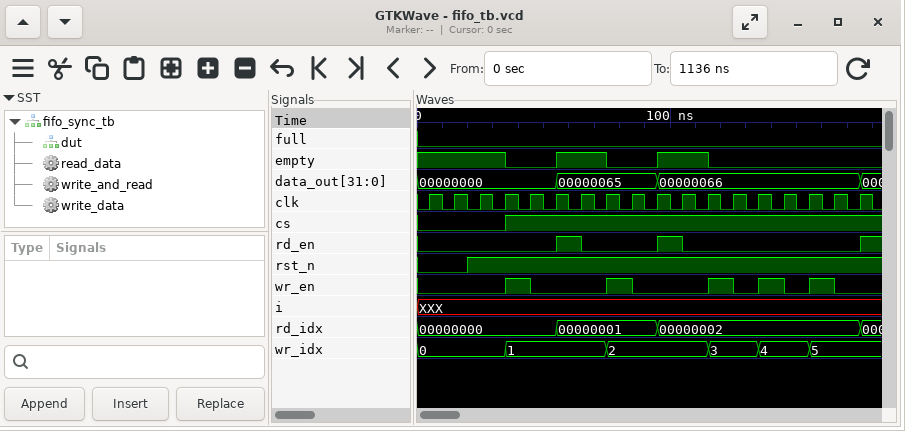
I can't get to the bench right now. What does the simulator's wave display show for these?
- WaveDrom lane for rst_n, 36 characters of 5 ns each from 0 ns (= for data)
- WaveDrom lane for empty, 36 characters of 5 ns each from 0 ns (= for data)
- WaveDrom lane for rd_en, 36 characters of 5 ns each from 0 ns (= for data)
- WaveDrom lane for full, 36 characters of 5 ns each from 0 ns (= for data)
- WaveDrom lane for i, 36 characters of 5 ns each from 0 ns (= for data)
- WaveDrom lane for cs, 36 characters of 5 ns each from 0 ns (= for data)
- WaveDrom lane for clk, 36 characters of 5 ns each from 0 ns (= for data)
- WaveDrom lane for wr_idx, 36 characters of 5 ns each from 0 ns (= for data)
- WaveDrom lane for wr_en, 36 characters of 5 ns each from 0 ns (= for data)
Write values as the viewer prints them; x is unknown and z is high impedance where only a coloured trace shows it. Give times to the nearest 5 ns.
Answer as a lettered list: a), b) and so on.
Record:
a) {name: 'rst_n', wave: '0...1...............................'}
b) {name: 'empty', wave: '1......0...1...0...1...0............'}
c) {name: 'rd_en', wave: '0..........1.0.....1.0.............1'}
d) {name: 'full', wave: '0...................................'}
e) {name: 'i', wave: 'x...................................'}
f) {name: 'cs', wave: '0......1............................'}
g) {name: 'clk', wave: '010101010101010101010101010101010101'}
h) {name: 'wr_idx', wave: '=......=.......=.......=...=...=....', data: '0 1 2 3 4 5'}
i) {name: 'wr_en', wave: '0......1.0.....1.0.....1.0.1.0.1.0..'}
